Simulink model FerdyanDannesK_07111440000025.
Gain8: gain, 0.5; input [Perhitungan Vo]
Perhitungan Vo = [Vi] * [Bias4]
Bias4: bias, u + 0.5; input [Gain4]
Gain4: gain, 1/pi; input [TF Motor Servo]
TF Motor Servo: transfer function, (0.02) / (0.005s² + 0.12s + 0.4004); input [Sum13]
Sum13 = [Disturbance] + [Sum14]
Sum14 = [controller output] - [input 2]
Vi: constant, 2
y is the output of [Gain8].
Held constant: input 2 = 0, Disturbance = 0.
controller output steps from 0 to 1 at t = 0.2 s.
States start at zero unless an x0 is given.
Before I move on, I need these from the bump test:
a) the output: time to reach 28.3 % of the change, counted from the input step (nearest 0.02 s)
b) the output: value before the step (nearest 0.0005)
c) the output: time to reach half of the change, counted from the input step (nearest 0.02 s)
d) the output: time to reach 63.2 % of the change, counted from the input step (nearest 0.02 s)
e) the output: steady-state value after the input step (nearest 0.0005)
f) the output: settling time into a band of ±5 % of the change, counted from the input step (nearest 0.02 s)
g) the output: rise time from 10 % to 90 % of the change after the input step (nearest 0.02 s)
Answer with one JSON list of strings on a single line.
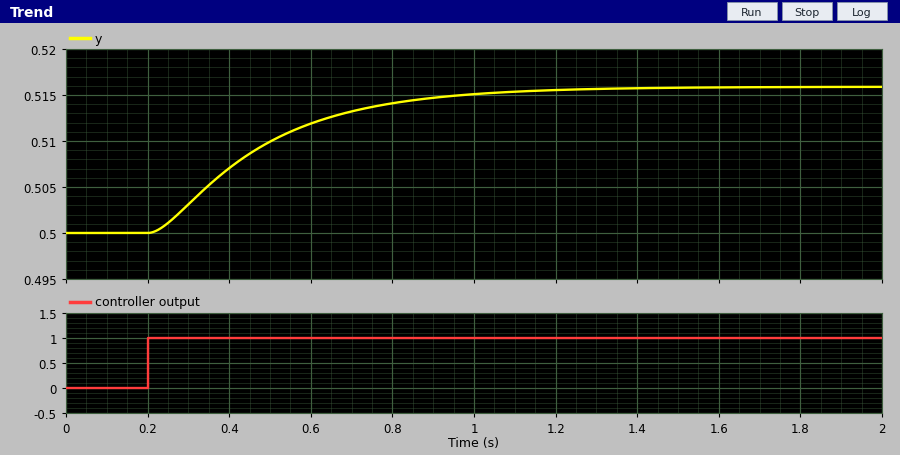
["0.14 s", "0.5000", "0.22 s", "0.30 s", "0.5160", "0.80 s", "0.56 s"]
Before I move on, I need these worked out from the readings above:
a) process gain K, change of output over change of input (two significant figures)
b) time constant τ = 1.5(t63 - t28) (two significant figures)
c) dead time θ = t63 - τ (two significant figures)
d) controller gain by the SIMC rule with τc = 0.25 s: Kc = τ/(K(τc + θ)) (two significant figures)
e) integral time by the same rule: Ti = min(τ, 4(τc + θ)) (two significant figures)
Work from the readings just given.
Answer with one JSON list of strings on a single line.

["0.016", "0.24 s", "0.060 s", "48", "0.24 s"]
